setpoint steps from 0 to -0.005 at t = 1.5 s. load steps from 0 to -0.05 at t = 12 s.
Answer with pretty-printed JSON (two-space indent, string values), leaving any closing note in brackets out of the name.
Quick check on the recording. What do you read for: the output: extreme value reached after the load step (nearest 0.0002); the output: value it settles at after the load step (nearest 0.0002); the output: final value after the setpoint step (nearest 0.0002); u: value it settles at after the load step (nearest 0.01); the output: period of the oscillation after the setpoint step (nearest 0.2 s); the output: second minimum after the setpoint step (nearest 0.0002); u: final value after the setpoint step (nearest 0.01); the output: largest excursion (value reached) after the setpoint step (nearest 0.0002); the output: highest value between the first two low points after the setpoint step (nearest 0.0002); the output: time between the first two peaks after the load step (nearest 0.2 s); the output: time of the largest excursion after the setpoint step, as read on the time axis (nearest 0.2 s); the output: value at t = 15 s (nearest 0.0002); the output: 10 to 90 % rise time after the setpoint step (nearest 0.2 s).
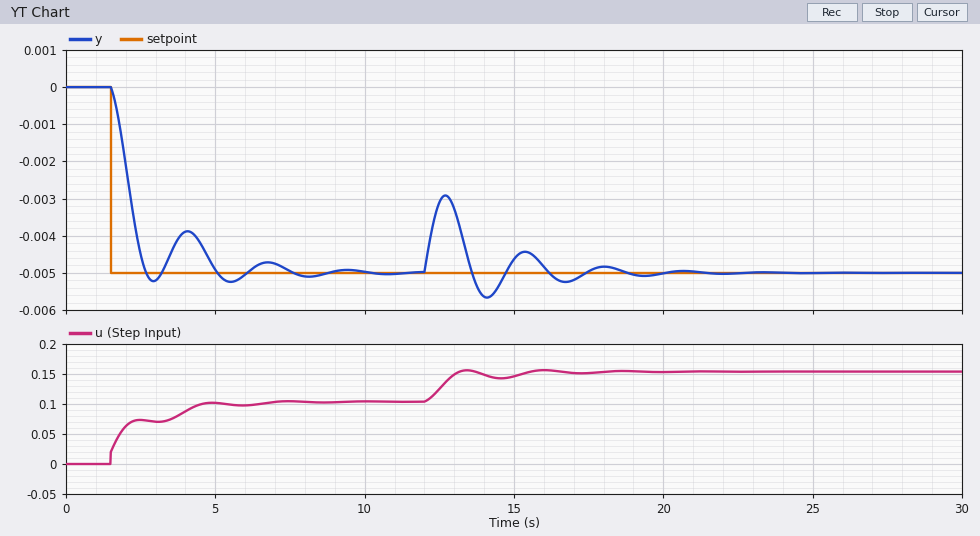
{
  "the output: extreme value reached after the load step": "-0.0030",
  "the output: value it settles at after the load step": "-0.0050",
  "the output: final value after the setpoint step": "-0.0050",
  "u: value it settles at after the load step": "0.15",
  "the output: period of the oscillation after the setpoint step": "2.6 s",
  "the output: second minimum after the setpoint step": "-0.0052",
  "u: final value after the setpoint step": "0.10",
  "the output: largest excursion (value reached) after the setpoint step": "-0.0052",
  "the output: highest value between the first two low points after the setpoint step": "-0.0038",
  "the output: time between the first two peaks after the load step": "2.6 s",
  "the output: time of the largest excursion after the setpoint step, as read on the time axis": "5.6 s",
  "the output: value at t = 15 s": "-0.0046",
  "the output: 10 to 90 % rise time after the setpoint step": "0.8 s"
}
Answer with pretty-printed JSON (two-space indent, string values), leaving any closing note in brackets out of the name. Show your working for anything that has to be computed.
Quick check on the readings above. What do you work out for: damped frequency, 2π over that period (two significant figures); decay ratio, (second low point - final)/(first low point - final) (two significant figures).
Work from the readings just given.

{
  "damped frequency, 2π over that period": "2π / 2.6 = 2.4 rad/s",
  "decay ratio, (second low point - final)/(first low point - final)": "(-0.0052 - (-0.005)) / (-0.0052 - (-0.005)) = 1.0"
}
